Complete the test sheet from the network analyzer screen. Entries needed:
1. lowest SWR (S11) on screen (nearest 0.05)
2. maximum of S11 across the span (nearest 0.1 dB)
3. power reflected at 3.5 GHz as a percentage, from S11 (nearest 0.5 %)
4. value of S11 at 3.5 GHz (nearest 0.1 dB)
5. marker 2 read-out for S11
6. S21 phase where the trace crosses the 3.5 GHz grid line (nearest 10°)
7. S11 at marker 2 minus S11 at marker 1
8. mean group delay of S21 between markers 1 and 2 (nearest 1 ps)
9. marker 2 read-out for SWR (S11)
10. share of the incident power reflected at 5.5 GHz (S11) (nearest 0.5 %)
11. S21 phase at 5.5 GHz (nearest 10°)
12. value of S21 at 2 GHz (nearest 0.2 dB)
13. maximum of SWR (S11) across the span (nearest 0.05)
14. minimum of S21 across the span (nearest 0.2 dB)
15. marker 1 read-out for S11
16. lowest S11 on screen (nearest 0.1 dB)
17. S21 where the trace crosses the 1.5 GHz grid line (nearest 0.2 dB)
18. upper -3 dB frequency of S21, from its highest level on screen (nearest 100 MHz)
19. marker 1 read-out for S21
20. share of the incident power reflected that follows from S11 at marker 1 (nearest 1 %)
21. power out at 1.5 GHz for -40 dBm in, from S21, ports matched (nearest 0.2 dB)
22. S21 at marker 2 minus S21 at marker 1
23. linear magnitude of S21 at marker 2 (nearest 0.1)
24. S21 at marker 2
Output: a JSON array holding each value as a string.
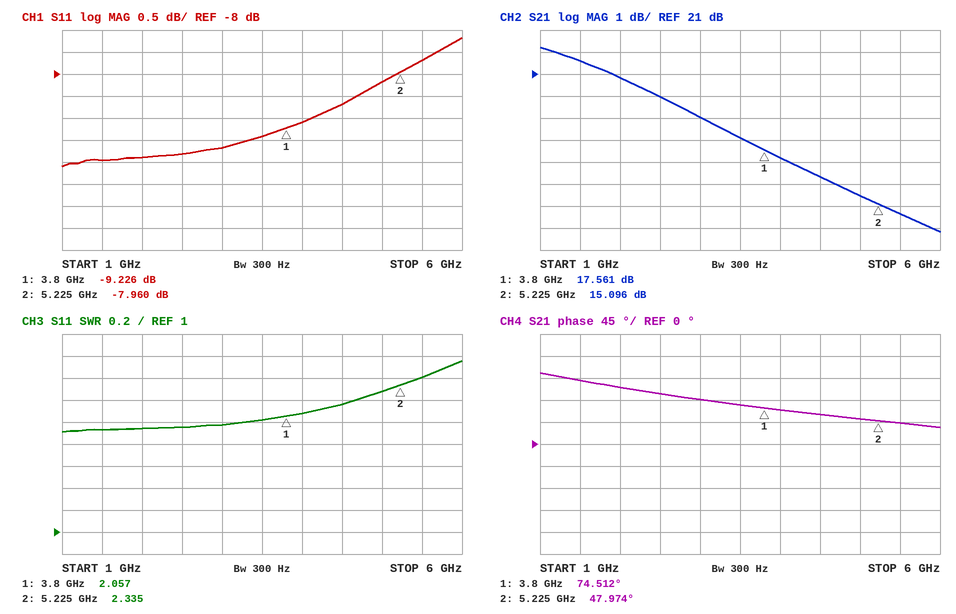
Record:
["1.90", "-7.2 dB", "11.5 %", "-9.4 dB", "-7.960 dB", "80°", "1.266 dB", "52 ps", "2.335", "17.0 %", "40°", "20.8 dB", "2.55", "13.8 dB", "-9.226 dB", "-10.1 dB", "21.6 dB", "2.9 GHz", "17.561 dB", "12 %", "-18.4 dBm", "-2.465 dB", "5.7", "15.096 dB"]
